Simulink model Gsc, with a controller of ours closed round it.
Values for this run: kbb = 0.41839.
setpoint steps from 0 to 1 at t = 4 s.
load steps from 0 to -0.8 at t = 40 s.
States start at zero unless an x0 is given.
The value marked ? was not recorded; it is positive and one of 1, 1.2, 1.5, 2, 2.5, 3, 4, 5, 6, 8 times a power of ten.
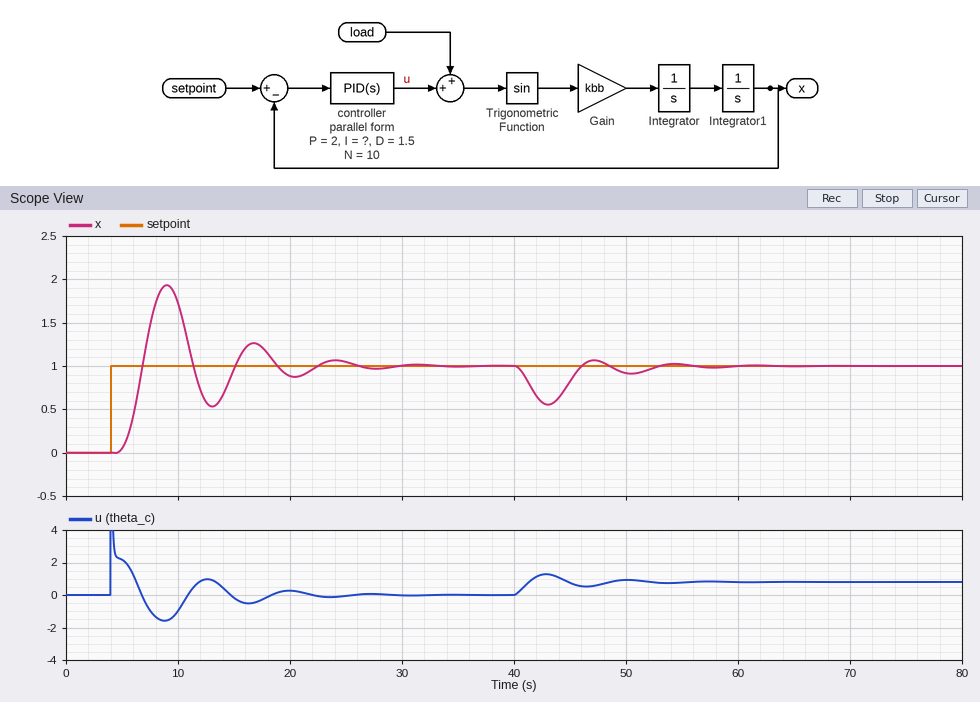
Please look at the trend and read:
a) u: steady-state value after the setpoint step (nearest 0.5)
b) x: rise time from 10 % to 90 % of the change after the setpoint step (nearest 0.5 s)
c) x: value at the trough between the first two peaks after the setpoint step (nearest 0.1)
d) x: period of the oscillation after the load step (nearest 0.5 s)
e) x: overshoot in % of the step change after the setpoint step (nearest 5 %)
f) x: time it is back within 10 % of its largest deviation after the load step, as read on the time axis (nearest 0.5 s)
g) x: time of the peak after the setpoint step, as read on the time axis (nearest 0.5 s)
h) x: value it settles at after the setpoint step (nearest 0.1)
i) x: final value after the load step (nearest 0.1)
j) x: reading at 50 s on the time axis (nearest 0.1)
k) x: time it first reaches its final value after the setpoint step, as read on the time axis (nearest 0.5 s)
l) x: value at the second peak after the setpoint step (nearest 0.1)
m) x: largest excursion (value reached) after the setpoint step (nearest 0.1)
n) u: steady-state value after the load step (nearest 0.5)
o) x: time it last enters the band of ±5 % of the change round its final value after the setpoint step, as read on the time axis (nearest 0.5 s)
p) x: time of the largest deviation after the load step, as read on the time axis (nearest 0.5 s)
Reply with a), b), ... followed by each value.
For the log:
a) 0.0
b) 1.5 s
c) 0.5
d) 7.5 s
e) 95 %
f) 52.0 s
g) 9.0 s
h) 1.0
i) 1.0
j) 0.9
k) 7.0 s
l) 1.3
m) 1.9
n) 1.0
o) 25.0 s
p) 43.0 s
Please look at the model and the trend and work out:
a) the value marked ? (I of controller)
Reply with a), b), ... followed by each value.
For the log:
a) 0.5
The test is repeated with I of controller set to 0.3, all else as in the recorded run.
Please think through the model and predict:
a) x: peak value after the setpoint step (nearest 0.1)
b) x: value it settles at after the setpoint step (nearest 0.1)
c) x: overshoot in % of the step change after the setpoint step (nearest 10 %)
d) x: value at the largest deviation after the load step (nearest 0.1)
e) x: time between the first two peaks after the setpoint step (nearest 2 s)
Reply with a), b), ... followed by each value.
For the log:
a) 1.7
b) 1.0
c) 70 %
d) 0.5
e) 8 s
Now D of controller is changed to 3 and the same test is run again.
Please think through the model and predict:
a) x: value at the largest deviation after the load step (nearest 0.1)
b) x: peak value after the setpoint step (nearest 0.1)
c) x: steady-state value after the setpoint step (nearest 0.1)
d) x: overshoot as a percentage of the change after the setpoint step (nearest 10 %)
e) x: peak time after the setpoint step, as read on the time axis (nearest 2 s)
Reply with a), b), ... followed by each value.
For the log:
a) 0.7
b) 1.5
c) 1.0
d) 50 %
e) 10 s
